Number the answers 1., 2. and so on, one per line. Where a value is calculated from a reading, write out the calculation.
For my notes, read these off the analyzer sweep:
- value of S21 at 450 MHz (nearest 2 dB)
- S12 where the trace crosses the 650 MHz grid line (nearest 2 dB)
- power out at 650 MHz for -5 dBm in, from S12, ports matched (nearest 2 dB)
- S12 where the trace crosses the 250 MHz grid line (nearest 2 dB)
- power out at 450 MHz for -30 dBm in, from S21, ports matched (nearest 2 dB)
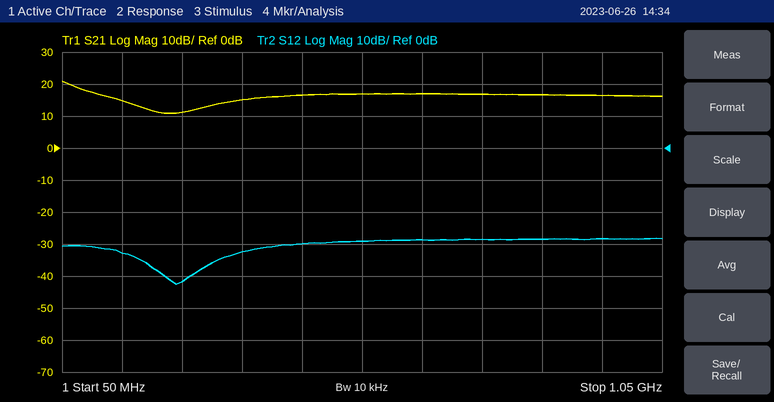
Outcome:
1. 16 dB
2. -28 dB
3. -5 dBm + (-28 dB) = -34 dBm
4. -42 dB
5. -30 dBm + (16 dB) = -14 dBm
